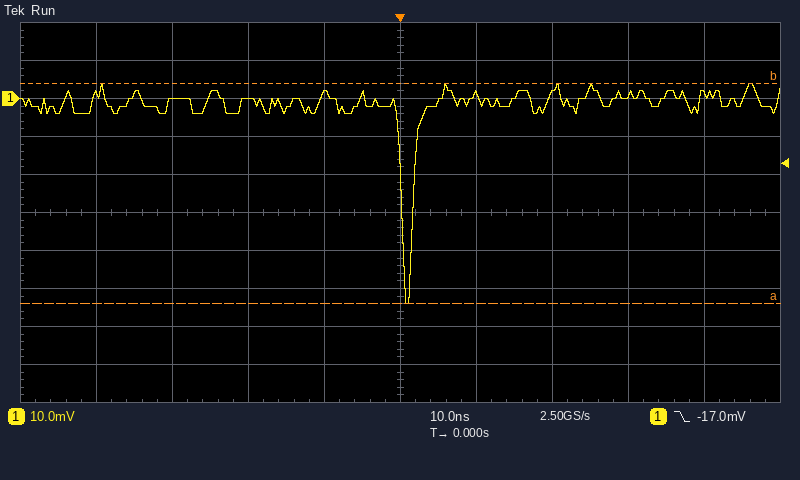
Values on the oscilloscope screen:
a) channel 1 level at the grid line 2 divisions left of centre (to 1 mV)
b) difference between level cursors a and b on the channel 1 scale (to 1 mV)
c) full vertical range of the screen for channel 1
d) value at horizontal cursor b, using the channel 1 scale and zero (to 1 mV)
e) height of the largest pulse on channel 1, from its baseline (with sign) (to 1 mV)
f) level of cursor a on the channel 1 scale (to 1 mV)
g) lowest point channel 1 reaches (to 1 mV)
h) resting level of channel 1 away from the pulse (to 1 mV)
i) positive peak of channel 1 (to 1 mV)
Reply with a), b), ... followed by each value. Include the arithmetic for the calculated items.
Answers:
a) 0 mV
b) 58 mV
c) 100 mV
d) 4 mV
e) -54 mV − (-1 mV) = -53 mV
f) -54 mV
g) -54 mV
h) -1 mV
i) 4 mV
